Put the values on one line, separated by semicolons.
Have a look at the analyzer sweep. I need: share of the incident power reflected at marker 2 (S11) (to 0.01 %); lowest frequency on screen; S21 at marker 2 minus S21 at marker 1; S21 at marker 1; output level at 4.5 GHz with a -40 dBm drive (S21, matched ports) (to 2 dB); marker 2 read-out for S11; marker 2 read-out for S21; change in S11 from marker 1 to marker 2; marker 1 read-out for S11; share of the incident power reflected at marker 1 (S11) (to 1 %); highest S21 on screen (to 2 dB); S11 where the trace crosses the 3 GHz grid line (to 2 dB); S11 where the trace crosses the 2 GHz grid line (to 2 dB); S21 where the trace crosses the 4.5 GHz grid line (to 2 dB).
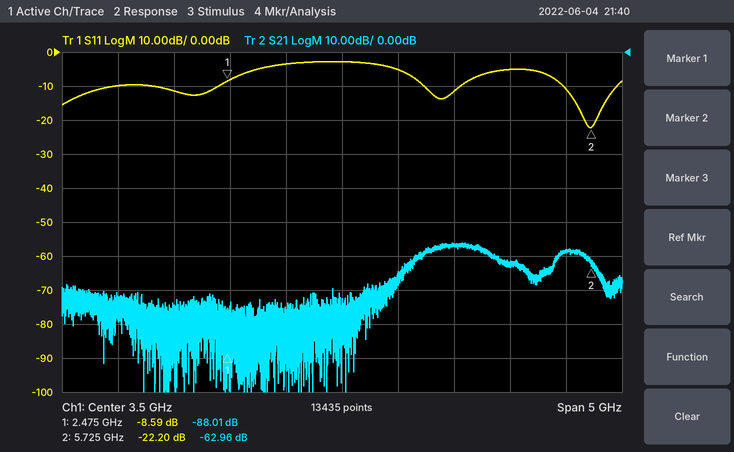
0.60 %; 1 GHz; 25.05 dB; -88.01 dB; -96 dBm; -22.20 dB; -62.96 dB; -13.61 dB; -8.59 dB; 14 %; -56 dB; -4 dB; -12 dB; -56 dB
